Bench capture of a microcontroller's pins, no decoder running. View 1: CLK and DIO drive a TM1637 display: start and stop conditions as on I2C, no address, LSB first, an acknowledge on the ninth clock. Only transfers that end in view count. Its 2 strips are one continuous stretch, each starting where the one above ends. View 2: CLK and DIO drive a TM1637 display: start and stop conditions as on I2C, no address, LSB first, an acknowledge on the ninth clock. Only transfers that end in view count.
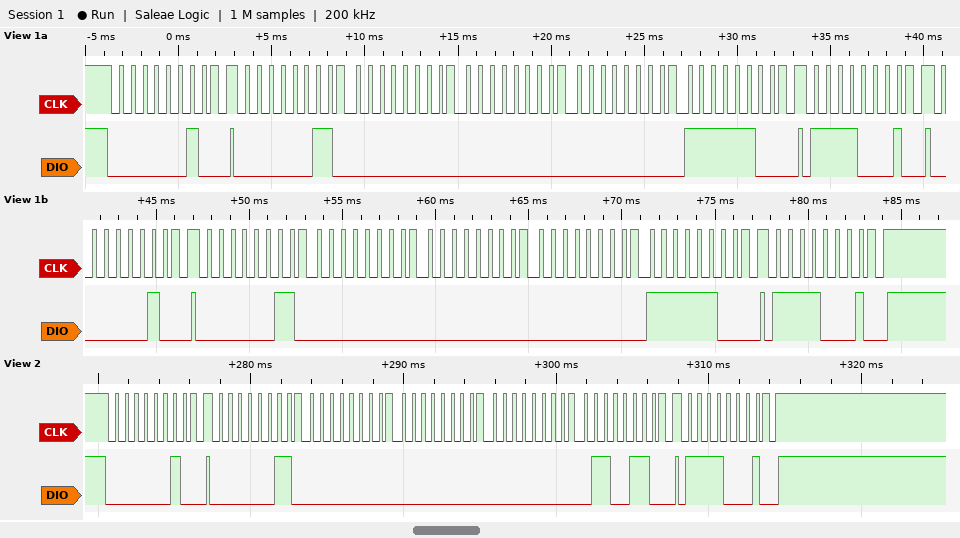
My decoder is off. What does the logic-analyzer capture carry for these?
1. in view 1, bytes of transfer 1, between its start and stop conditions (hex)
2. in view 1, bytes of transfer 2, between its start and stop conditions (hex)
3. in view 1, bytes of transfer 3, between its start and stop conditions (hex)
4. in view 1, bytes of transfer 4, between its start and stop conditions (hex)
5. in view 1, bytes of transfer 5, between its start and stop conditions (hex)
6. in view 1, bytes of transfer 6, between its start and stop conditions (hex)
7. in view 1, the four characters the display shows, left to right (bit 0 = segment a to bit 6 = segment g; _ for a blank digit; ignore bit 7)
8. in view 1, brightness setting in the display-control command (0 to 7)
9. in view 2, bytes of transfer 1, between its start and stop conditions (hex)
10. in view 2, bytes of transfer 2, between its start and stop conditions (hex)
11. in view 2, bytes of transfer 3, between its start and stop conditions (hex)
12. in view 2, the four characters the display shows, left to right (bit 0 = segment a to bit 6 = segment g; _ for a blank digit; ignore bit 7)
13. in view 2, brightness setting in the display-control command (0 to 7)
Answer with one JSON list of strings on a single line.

["40", "C0 00 00 00 3F", "8F", "40", "C0 00 00 00 3F", "8F", "___0", "7", "40", "C0 00 00 00 66", "8F", "___4", "7"]
